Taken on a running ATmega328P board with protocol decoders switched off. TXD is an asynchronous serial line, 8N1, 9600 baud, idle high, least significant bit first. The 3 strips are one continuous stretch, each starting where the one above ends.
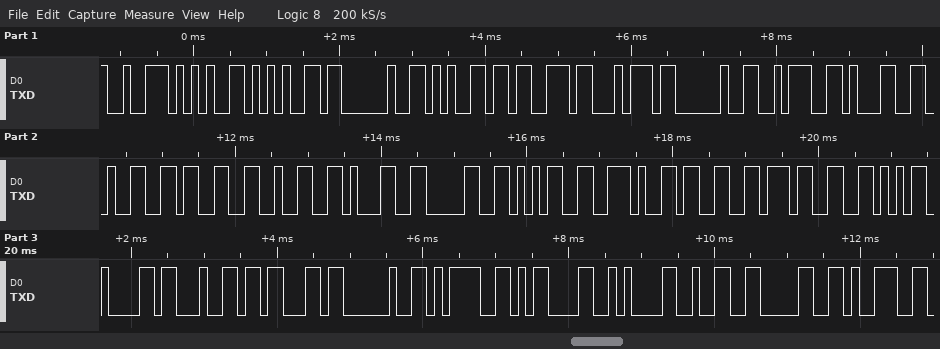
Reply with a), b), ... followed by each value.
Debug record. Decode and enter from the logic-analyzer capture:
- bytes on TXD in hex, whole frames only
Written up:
a) 72 65 65 20 65 73 74 20 3A 31 32 33 32 31 30 35 2E 33 37 56 61 64 63 20 3D 0D 0A 32 30 39
